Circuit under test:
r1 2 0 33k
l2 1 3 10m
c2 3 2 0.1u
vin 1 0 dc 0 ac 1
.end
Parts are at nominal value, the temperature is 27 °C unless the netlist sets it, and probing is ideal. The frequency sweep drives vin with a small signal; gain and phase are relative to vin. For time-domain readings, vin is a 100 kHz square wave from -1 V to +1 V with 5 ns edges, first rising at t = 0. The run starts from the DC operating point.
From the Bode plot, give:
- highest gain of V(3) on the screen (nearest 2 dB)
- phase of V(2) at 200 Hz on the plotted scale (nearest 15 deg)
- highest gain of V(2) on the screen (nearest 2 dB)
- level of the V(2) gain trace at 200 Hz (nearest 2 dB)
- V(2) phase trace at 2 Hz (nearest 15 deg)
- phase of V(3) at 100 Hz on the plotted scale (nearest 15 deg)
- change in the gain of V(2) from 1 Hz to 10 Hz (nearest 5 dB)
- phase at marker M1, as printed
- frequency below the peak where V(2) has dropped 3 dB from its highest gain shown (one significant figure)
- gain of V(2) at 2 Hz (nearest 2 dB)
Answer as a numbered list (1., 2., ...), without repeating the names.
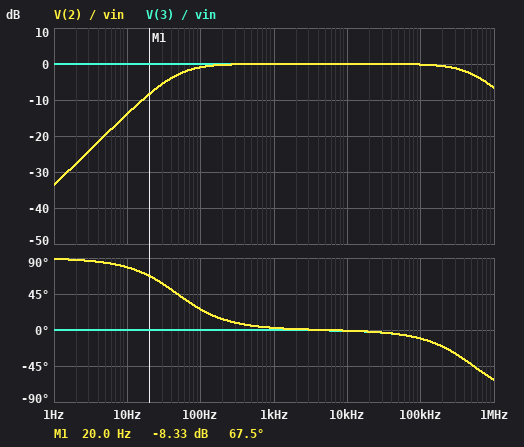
1. 0 dB
2. 15 deg
3. 0 dB
4. 0 dB
5. 90 deg
6. 0 deg
7. 20 dB
8. 67.5 deg
9. 50 Hz
10. -28 dB
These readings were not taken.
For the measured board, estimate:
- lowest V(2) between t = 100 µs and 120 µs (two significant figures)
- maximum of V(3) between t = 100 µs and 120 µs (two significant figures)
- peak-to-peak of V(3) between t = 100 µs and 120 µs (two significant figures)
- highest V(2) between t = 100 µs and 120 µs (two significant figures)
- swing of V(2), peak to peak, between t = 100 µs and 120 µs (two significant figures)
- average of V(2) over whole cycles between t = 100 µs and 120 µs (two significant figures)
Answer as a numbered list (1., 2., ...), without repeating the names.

1. -36 mV
2. 1.0 V
3. 2.0 V
4. 2.0 V
5. 2.0 V
6. 970 mV
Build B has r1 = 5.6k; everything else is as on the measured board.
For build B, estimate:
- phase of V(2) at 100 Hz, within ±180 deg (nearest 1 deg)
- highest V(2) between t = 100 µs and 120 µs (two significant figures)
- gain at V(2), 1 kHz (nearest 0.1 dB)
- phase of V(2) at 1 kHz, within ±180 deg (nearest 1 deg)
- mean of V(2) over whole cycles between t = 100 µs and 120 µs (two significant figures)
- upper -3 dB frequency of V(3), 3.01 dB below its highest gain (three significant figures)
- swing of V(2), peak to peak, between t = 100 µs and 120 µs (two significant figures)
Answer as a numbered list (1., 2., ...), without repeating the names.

1. 71 deg
2. 1.7 V
3. -0.3 dB
4. 15 deg
5. 830 mV
6. 88.9 kHz
7. 1.8 V
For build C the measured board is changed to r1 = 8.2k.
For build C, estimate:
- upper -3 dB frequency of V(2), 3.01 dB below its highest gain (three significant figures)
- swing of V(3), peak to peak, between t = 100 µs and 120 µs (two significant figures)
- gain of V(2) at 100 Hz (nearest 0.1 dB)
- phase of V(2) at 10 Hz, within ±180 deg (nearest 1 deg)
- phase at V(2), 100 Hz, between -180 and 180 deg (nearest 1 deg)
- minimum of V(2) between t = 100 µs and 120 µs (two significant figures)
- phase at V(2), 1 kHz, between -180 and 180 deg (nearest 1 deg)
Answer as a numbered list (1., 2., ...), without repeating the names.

1. 131 kHz
2. 1.9 V
3. -6.8 dB
4. 87 deg
5. 63 deg
6. -100 mV
7. 11 deg
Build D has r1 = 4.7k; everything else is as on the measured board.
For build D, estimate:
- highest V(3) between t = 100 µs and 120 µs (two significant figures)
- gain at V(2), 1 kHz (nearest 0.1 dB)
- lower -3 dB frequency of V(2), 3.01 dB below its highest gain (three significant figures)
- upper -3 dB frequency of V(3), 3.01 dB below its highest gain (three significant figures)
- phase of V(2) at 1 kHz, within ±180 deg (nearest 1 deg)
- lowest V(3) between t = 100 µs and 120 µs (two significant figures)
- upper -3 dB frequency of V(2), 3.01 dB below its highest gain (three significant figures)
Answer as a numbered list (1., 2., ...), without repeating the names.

1. 830 mV
2. -0.4 dB
3. 337 Hz
4. 74.5 kHz
5. 18 deg
6. -820 mV
7. 75.1 kHz
